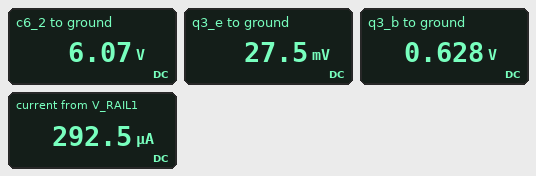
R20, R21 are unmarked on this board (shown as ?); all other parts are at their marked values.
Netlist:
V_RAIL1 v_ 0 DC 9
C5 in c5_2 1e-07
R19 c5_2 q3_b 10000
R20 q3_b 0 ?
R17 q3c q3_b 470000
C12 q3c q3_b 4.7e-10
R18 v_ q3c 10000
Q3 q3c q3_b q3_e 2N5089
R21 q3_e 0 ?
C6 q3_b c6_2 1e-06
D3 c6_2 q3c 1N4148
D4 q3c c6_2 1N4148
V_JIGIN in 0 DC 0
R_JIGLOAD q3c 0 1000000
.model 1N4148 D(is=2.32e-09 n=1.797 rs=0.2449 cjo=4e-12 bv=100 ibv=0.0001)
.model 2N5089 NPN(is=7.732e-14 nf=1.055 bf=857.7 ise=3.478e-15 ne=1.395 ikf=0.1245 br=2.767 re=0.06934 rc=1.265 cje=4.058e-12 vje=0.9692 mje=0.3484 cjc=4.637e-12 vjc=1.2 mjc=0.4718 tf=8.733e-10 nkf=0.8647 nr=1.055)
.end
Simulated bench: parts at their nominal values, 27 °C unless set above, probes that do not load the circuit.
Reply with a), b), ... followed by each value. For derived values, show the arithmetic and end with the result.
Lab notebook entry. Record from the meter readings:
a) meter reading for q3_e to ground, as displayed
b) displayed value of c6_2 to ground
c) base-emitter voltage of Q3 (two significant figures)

a) 27.5 mV
b) 6.07 V
c) 628 mV - 27.5 mV = 600 mV
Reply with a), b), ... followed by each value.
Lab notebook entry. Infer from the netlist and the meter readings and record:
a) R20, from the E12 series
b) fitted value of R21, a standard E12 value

a) 56 kΩ
b) 100 Ω
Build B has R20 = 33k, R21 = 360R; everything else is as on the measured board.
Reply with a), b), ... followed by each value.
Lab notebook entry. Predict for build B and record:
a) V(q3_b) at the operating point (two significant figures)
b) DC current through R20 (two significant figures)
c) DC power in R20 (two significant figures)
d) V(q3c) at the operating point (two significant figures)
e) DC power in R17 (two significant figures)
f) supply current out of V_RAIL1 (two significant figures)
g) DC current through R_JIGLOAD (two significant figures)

a) 550 mV
b) 17 µA
c) 9.2 µW
d) 8.4 V
e) 130 µW
f) 56 µA
g) 8.4 µA
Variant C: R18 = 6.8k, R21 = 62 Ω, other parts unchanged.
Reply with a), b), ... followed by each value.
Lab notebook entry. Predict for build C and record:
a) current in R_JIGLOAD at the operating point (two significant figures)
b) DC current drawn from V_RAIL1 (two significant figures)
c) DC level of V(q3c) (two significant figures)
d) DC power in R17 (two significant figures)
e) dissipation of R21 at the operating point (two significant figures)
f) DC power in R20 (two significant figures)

a) 6.2 µA
b) 410 µA
c) 6.2 V
d) 66 µW
e) 9.6 µW
f) 7.2 µW
